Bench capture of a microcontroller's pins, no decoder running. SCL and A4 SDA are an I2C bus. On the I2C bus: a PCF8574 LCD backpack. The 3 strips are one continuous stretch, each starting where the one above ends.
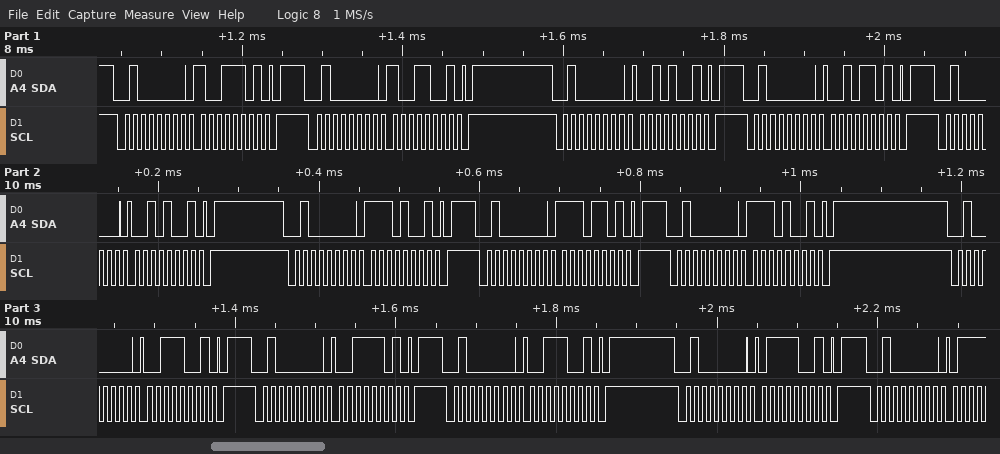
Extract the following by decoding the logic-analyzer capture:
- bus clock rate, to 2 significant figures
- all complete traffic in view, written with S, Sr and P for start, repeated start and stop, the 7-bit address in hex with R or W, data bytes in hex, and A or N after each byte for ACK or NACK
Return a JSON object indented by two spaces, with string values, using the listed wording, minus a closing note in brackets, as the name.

{
  "bus clock rate, to 2 significant figures": "100 kHz",
  "all complete traffic in view, written with S, Sr and P for start, repeated start and stop, the 7-bit address in hex with R or W, data bytes in hex, and A or N after each byte for ACK or NACK": "S 20W A 9D A P S 20W A 99 A P S 20W A 29 A P S 20W A 2D A P S 20W A 29 A P S 20W A E9 A P S 20W A ED A P S 20W A E9 A P S 20W A 39 A P S 20W A 3D A P S 20W A 39 A P S 20W A 79 A P S 20W A"
}
